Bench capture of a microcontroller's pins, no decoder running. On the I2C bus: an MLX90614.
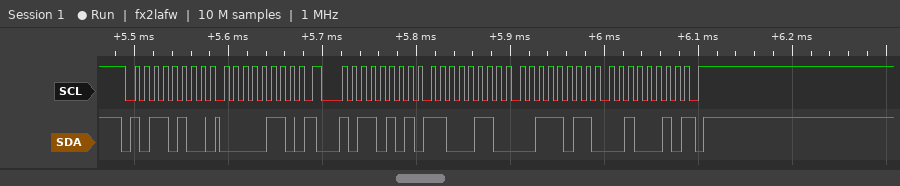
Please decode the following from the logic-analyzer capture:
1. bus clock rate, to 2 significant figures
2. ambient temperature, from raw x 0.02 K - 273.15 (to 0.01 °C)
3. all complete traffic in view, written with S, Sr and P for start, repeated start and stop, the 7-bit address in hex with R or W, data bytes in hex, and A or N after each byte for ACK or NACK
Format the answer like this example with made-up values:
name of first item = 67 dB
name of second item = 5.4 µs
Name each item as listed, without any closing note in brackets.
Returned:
bus clock rate, to 2 significant figures = 100 kHz
ambient temperature, from raw x 0.02 K - 273.15 = 32.89 °C
all complete traffic in view, written with S, Sr and P for start, repeated start and stop, the 7-bit address in hex with R or W, data bytes in hex, and A or N after each byte for ACK or NACK = S 5AW A 06 A Sr 5AR A C6 A 3B A 22 N P
